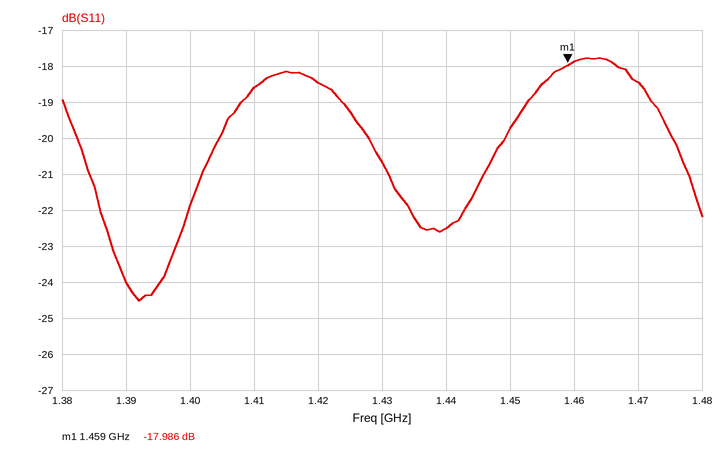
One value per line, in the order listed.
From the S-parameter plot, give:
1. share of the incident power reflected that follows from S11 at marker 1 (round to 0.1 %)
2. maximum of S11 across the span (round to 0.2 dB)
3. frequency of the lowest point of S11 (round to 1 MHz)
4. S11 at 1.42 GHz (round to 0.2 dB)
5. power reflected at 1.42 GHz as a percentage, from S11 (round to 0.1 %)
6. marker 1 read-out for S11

1.6 %
-17.8 dB
1.392 GHz
-18.4 dB
1.4 %
-17.986 dB
